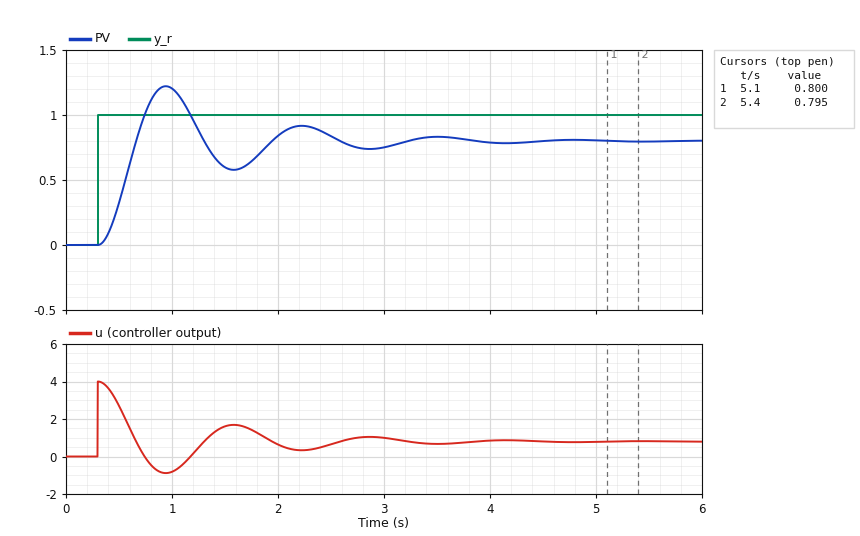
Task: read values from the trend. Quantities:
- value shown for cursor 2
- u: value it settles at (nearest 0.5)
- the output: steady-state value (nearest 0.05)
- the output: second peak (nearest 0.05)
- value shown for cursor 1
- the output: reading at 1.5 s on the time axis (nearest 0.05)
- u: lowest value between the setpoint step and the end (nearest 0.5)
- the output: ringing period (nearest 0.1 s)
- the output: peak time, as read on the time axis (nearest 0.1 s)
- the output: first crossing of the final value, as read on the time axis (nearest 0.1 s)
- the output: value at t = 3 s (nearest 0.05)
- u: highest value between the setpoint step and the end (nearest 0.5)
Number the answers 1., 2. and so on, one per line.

1. 0.795
2. 1.0
3. 0.80
4. 0.90
5. 0.800
6. 0.60
7. -1.0
8. 1.3 s
9. 0.9 s
10. 0.7 s
11. 0.75
12. 4.0
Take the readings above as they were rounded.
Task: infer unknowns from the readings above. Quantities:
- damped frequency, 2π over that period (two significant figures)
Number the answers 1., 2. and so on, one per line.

1. 4.8 rad/s
